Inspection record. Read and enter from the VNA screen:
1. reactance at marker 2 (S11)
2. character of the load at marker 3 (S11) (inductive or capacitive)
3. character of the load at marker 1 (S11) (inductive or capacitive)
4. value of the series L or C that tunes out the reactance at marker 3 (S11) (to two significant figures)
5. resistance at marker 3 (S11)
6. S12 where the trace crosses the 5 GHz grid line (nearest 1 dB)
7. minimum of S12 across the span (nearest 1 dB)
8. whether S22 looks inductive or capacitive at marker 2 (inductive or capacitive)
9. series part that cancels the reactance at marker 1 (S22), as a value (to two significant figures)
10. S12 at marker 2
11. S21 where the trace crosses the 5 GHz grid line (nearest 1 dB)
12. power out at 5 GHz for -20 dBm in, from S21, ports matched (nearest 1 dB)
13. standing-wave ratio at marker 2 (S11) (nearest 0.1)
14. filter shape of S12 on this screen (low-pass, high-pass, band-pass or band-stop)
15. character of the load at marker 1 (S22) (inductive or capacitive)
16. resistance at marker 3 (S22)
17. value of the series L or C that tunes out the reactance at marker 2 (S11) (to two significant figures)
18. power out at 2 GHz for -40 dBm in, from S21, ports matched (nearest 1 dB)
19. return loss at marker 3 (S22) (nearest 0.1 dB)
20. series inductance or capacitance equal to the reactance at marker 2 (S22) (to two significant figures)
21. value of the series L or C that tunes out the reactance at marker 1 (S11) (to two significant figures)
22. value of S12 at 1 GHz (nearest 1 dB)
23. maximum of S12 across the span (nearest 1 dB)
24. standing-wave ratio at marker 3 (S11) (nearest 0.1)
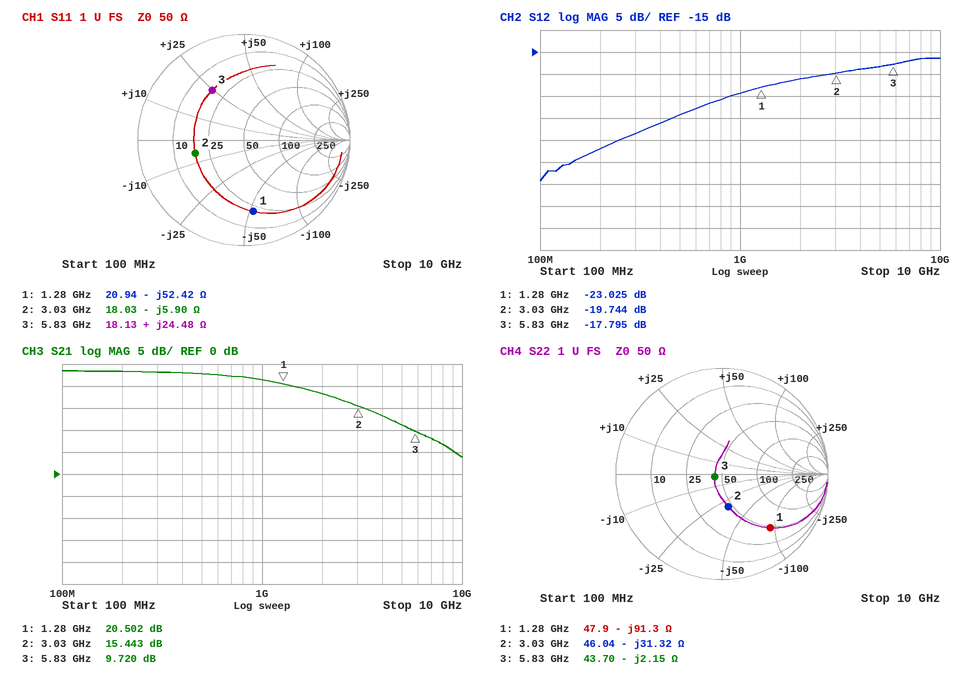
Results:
-5.90 Ω
inductive
capacitive
1.1 pF
18.13 Ω
-18 dB
-44 dB
capacitive
11 nH
-19.744 dB
11 dB
-9 dBm
2.8
high-pass
capacitive
43.70 Ω
310 pH
-22 dBm
23.0 dB
1.7 pF
6.5 nH
-24 dB
-16 dB
3.5
